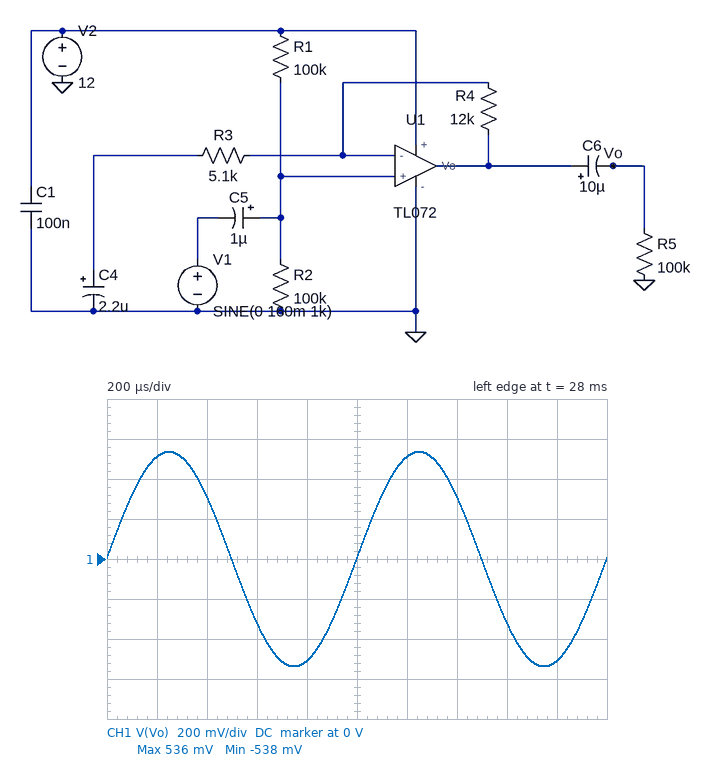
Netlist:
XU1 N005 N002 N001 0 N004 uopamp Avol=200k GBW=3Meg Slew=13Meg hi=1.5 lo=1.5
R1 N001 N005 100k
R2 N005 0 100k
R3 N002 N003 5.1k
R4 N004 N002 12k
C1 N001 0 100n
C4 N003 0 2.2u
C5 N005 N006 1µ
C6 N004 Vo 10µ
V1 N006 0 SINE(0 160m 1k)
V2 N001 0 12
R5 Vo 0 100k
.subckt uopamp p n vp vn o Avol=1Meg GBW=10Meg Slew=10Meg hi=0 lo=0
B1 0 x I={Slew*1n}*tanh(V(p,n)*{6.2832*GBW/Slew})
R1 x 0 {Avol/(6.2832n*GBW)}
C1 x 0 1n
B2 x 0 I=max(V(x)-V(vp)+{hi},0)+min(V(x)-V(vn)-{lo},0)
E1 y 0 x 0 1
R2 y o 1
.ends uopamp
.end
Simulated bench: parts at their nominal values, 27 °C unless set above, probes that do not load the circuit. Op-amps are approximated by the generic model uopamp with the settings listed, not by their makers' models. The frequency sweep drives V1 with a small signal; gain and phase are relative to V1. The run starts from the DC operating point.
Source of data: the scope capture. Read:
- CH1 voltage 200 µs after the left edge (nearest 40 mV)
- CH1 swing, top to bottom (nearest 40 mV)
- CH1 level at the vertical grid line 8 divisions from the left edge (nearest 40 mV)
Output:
520 mV
1.08 V
-320 mV
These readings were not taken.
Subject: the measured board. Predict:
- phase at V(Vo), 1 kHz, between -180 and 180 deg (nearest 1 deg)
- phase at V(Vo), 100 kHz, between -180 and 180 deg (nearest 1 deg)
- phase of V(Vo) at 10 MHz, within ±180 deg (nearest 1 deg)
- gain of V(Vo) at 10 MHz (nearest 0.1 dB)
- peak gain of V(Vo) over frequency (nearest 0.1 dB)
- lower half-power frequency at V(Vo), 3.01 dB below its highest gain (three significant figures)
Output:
1 deg
-6 deg
-85 deg
-10.5 dB
10.5 dB
13.7 Hz
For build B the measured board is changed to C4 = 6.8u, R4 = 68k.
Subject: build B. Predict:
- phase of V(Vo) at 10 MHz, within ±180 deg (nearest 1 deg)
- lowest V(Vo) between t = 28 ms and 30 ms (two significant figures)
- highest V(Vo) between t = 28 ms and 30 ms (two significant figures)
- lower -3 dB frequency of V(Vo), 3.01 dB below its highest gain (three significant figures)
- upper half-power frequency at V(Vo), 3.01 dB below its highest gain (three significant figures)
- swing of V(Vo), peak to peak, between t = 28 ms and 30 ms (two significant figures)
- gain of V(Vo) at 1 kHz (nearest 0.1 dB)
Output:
-89 deg
-2.3 V
2.3 V
6.07 Hz
209 kHz
4.6 V
23.1 dB
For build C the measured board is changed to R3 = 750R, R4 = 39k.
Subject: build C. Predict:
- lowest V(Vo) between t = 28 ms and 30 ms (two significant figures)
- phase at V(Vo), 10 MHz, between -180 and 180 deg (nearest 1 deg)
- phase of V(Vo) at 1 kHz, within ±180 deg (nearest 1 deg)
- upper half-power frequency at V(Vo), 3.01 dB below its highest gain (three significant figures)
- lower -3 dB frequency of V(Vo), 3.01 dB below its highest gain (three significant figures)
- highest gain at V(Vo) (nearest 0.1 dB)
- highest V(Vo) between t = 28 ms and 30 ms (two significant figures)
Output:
-4.5 V
-90 deg
5 deg
56.7 kHz
96.3 Hz
34.5 dB
4.5 V
